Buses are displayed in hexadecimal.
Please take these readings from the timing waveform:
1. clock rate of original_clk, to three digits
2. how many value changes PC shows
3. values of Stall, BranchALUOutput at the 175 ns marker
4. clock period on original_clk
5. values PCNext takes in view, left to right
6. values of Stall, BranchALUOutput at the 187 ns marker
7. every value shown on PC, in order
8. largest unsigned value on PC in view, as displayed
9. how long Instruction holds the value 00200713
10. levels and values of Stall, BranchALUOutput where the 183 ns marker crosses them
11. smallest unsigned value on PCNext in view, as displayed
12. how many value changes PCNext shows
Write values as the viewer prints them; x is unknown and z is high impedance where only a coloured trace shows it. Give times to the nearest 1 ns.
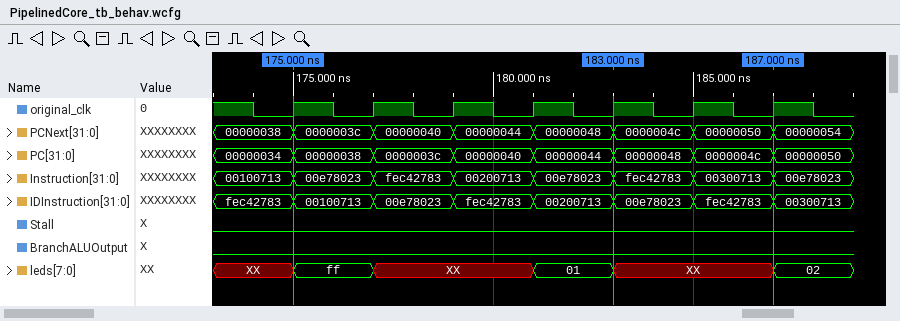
500 MHz
7
Stall=0, BranchALUOutput=0
2 ns
00000038, 0000003c, 00000040, 00000044, 00000048, 0000004c, 00000050, 00000054
Stall=0, BranchALUOutput=0
00000034, 00000038, 0000003c, 00000040, 00000044, 00000048, 0000004c, 00000050
00000050
2 ns
Stall=0, BranchALUOutput=0
00000038
7
